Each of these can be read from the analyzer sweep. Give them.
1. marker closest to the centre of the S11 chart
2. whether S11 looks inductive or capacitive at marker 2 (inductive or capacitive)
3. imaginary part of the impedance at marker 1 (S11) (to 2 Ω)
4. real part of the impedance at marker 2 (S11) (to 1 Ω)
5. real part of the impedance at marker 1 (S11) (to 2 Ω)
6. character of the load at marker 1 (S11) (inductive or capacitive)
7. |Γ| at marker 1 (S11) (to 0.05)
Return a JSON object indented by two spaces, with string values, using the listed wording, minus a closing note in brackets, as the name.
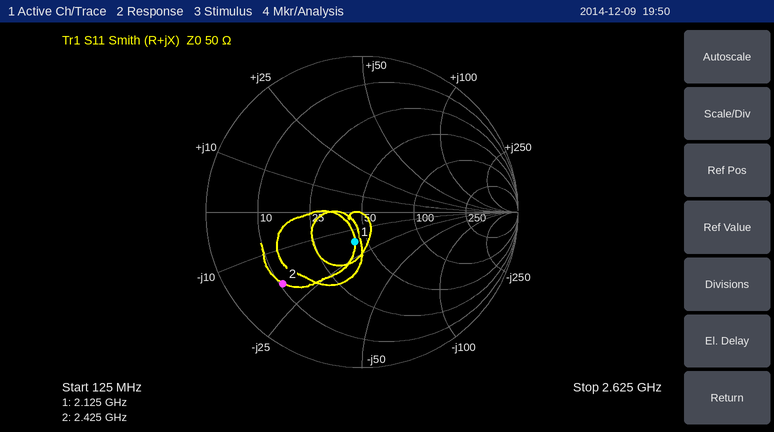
{
  "marker closest to the centre of the S11 chart": "marker 1",
  "whether S11 looks inductive or capacitive at marker 2": "capacitive",
  "imaginary part of the impedance at marker 1 (S11)": "-16 Ω",
  "real part of the impedance at marker 2 (S11)": "11 Ω",
  "real part of the impedance at marker 1 (S11)": "42 Ω",
  "character of the load at marker 1 (S11)": "capacitive",
  "|Γ| at marker 1 (S11)": "0.20"
}
